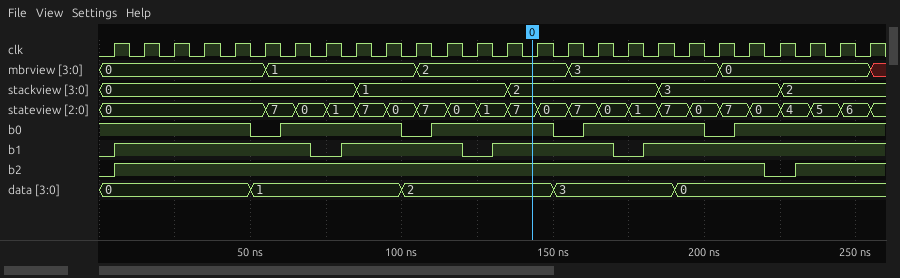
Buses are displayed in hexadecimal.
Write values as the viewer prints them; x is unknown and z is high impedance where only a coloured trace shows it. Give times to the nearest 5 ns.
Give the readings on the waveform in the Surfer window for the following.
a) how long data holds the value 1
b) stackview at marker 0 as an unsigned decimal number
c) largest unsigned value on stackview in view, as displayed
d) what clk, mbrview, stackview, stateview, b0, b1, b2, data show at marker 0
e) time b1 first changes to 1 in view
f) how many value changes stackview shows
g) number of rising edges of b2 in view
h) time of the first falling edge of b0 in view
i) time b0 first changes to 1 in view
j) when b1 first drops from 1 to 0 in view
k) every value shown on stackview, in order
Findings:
50 ns
2
3
clk=0, mbrview=2, stackview=2, stateview=7, b0=1, b1=1, b2=1, data=2
5 ns
4
2
50 ns
60 ns
70 ns
0, 1, 2, 3, 2
